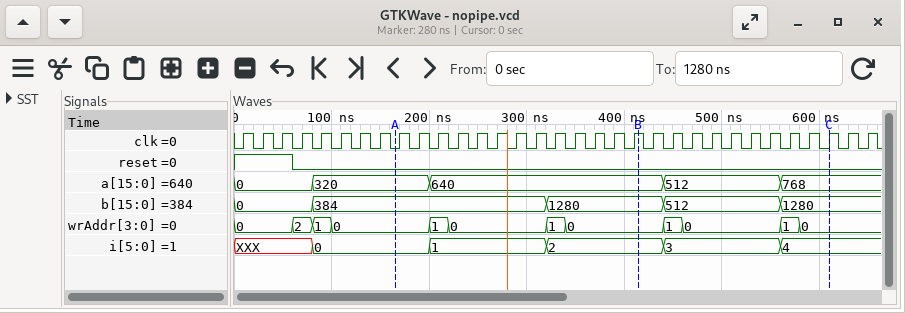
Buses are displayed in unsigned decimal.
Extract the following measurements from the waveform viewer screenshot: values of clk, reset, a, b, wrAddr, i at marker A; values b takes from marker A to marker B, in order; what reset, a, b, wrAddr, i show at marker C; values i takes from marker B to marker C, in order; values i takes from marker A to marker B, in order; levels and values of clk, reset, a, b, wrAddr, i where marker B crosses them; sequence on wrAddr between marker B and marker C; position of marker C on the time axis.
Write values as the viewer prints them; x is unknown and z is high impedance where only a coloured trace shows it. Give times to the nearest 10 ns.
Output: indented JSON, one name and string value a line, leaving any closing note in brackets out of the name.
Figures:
{
  "values of clk, reset, a, b, wrAddr, i at marker A": "clk=0, reset=0, a=320, b=384, wrAddr=0, i=0",
  "values b takes from marker A to marker B, in order": "384, 1280",
  "what reset, a, b, wrAddr, i show at marker C": "reset=0, a=768, b=1280, wrAddr=0, i=4",
  "values i takes from marker B to marker C, in order": "2, 3, 4",
  "values i takes from marker A to marker B, in order": "0, 1, 2",
  "levels and values of clk, reset, a, b, wrAddr, i where marker B crosses them": "clk=1, reset=0, a=640, b=1280, wrAddr=0, i=2",
  "sequence on wrAddr between marker B and marker C": "0, 1, 0, 1, 0",
  "position of marker C on the time axis": "610 ns"
}
